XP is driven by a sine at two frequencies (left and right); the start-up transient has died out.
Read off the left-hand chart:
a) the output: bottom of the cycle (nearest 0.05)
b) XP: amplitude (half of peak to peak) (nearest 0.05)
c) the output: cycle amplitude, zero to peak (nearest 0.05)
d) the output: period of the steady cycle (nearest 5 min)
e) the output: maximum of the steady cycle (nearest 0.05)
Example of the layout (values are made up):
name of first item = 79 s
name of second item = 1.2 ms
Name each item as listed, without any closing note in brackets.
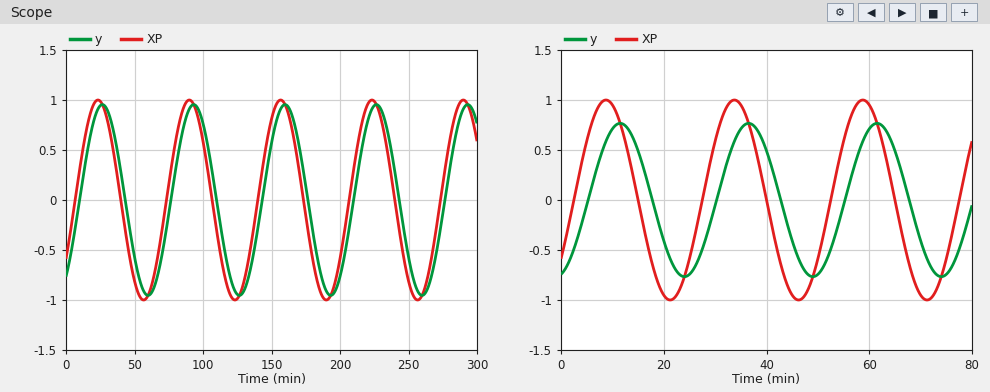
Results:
the output: bottom of the cycle = -0.95
XP: amplitude (half of peak to peak) = 1.00
the output: cycle amplitude, zero to peak = 0.95
the output: period of the steady cycle = 65 min
the output: maximum of the steady cycle = 0.95
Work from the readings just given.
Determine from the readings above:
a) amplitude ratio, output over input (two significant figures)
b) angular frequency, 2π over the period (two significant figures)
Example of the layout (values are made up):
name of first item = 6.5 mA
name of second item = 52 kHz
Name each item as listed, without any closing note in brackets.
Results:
amplitude ratio, output over input = 0.95
angular frequency, 2π over the period = 0.097 rad/min
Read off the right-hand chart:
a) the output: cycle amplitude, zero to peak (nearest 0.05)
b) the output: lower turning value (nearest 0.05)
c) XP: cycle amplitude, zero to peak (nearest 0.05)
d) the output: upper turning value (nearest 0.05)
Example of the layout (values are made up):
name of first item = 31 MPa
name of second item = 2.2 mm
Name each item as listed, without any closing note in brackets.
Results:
the output: cycle amplitude, zero to peak = 0.75
the output: lower turning value = -0.75
XP: cycle amplitude, zero to peak = 1.00
the output: upper turning value = 0.75
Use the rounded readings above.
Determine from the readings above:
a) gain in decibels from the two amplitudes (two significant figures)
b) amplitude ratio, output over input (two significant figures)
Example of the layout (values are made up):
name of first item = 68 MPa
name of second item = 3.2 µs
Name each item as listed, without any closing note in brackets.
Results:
gain in decibels from the two amplitudes = -2.5 dB
amplitude ratio, output over input = 0.75
